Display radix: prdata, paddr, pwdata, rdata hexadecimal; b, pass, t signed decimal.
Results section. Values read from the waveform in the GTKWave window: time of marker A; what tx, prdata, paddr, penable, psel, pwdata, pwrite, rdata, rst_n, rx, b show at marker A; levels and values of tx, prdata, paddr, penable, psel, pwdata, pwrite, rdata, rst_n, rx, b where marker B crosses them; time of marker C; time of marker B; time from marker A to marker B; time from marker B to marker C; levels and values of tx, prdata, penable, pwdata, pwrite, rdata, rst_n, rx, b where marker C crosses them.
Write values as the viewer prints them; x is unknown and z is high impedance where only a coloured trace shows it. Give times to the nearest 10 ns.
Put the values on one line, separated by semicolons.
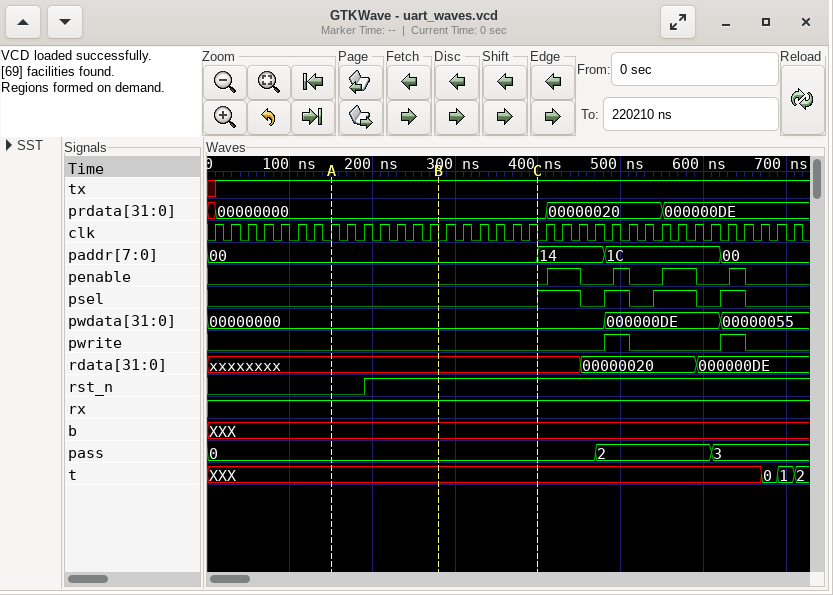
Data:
150 ns; tx=1, prdata=00000000, paddr=00, penable=0, psel=0, pwdata=00000000, pwrite=0, rdata=xxxxxxxx, rst_n=0, rx=1, b=XXX; tx=1, prdata=00000000, paddr=00, penable=0, psel=0, pwdata=00000000, pwrite=0, rdata=xxxxxxxx, rst_n=1, rx=1, b=XXX; 400 ns; 280 ns; 130 ns; 120 ns; tx=1, prdata=00000000, penable=0, pwdata=00000000, pwrite=0, rdata=xxxxxxxx, rst_n=1, rx=1, b=XXX
